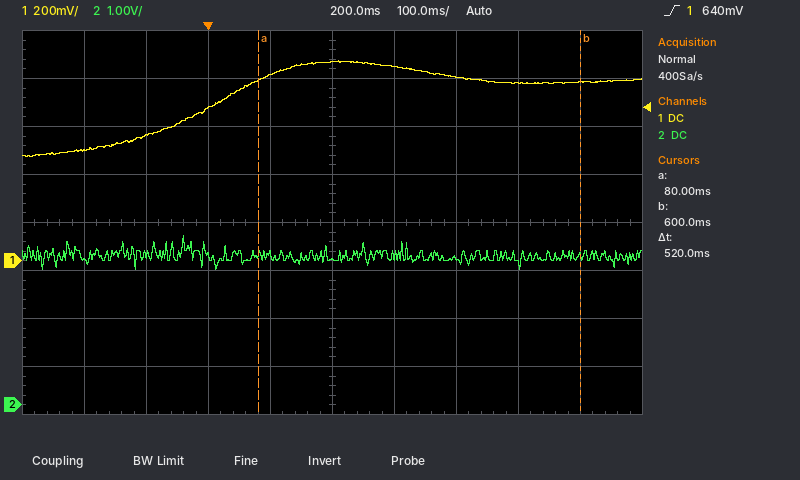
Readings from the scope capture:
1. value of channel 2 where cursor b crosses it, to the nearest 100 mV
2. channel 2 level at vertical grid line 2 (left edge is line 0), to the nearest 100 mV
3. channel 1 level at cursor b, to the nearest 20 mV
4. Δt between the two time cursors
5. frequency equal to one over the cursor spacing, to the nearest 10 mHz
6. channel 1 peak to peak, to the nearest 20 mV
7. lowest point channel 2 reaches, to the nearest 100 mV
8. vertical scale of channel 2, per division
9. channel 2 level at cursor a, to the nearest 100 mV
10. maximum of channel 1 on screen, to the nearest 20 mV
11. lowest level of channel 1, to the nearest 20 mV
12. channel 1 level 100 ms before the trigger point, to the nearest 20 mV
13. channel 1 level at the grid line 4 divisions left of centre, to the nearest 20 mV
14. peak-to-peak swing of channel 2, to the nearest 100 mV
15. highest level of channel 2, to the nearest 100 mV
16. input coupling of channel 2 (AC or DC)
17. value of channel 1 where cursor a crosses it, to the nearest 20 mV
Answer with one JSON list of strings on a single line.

["3.1 V", "3.1 V", "740 mV", "520 ms", "1.92 Hz", "400 mV", "2.8 V", "1 V", "3.1 V", "840 mV", "440 mV", "520 mV", "460 mV", "700 mV", "3.5 V", "DC", "760 mV"]
